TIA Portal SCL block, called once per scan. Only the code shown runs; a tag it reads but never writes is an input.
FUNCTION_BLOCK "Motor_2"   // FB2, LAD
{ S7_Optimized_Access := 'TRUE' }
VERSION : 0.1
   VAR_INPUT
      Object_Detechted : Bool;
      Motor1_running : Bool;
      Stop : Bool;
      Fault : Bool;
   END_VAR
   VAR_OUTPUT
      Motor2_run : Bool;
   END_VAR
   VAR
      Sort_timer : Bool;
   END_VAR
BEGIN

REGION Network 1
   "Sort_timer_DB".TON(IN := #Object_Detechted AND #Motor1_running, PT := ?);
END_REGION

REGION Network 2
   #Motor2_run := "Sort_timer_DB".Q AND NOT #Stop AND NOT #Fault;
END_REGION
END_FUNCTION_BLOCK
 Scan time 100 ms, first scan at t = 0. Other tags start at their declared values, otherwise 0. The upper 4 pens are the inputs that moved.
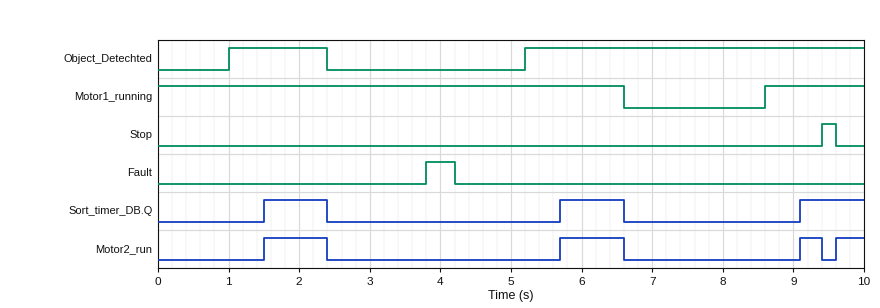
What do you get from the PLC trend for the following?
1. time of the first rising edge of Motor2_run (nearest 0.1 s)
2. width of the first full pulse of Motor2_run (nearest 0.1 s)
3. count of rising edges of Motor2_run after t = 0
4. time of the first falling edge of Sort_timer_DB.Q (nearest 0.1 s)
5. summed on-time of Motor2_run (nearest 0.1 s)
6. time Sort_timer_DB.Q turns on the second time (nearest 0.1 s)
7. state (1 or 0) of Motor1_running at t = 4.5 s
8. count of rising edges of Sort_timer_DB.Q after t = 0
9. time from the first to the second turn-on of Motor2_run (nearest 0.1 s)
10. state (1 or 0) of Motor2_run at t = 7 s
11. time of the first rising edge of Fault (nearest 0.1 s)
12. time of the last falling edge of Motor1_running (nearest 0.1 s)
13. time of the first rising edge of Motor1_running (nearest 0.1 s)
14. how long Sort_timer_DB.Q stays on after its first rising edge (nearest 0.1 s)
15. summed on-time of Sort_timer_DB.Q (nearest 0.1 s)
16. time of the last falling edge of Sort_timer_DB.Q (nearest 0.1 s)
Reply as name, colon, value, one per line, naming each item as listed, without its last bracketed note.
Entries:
time of the first rising edge of Motor2_run: 1.5 s
width of the first full pulse of Motor2_run: 0.9 s
count of rising edges of Motor2_run after t = 0: 4
time of the first falling edge of Sort_timer_DB.Q: 2.4 s
summed on-time of Motor2_run: 2.5 s
time Sort_timer_DB.Q turns on the second time: 5.7 s
state (1 or 0) of Motor1_running at t = 4.5 s: 1
count of rising edges of Sort_timer_DB.Q after t = 0: 3
time from the first to the second turn-on of Motor2_run: 4.2 s
state (1 or 0) of Motor2_run at t = 7 s: 0
time of the first rising edge of Fault: 3.8 s
time of the last falling edge of Motor1_running: 6.6 s
time of the first rising edge of Motor1_running: 8.6 s
how long Sort_timer_DB.Q stays on after its first rising edge: 0.9 s
summed on-time of Sort_timer_DB.Q: 2.7 s
time of the last falling edge of Sort_timer_DB.Q: 6.6 s
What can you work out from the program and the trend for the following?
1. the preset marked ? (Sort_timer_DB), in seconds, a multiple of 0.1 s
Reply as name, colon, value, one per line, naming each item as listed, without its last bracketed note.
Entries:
the preset marked ? (Sort_timer_DB), in seconds, a multiple of 0.1 s: 0.5 s
